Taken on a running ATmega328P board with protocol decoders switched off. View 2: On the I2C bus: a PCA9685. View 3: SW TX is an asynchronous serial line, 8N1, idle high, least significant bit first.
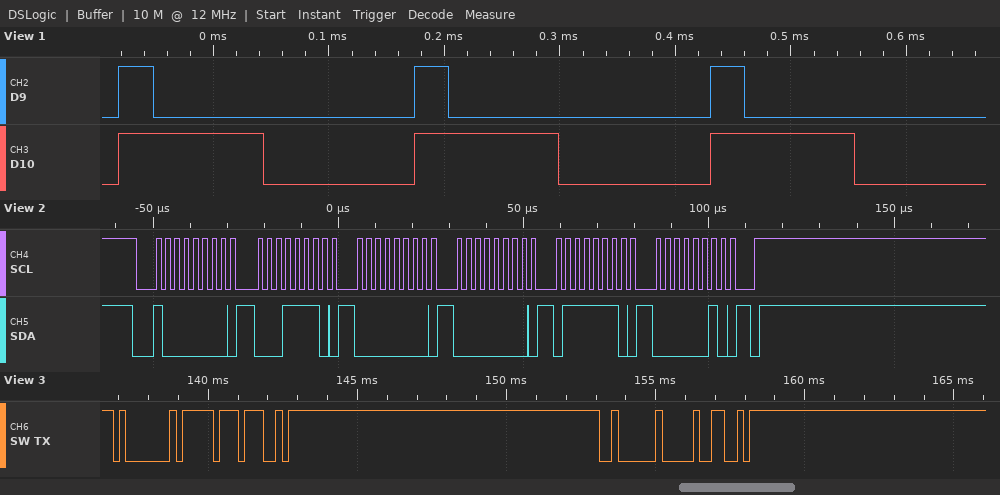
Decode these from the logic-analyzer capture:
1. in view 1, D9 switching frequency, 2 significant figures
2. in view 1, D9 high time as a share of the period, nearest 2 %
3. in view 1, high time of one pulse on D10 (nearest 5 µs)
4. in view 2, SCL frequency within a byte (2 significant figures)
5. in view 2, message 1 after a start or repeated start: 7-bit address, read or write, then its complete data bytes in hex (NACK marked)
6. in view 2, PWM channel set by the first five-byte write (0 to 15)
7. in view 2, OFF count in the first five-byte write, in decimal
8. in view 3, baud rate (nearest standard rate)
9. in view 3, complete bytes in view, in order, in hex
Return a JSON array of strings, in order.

["3.9 kHz", "12 %", "125 µs", "400 kHz", "0x40 write: 1E 00 00 7E 02", "6", "638", "4800 baud", "01 DF A7 02 90 FA"]
